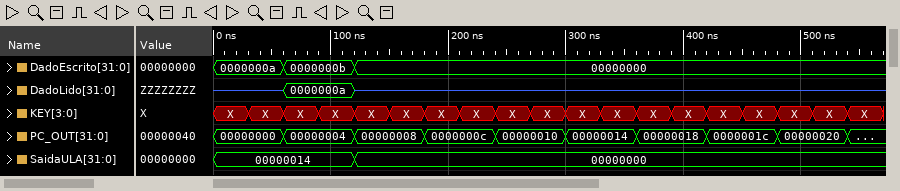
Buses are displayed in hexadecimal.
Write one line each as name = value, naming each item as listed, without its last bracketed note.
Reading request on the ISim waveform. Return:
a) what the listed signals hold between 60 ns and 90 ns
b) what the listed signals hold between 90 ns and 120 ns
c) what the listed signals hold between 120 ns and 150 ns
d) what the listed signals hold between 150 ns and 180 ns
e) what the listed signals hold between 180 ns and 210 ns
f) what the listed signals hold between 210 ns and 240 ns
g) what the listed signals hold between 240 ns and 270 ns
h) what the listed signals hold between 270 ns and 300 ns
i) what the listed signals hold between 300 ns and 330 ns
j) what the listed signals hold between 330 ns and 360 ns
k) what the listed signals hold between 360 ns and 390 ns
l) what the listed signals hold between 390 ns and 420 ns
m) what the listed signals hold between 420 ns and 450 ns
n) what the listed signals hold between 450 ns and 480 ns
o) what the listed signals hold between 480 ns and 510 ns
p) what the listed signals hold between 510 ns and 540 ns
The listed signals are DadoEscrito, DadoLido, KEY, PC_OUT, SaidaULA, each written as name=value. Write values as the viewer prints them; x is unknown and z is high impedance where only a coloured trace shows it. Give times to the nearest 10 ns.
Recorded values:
what the listed signals hold between 60 ns and 90 ns = DadoEscrito=0000000b, DadoLido=0000000a, KEY=X, PC_OUT=00000004, SaidaULA=00000014
what the listed signals hold between 90 ns and 120 ns = DadoEscrito=0000000b, DadoLido=0000000a, KEY=X, PC_OUT=00000004, SaidaULA=00000014
what the listed signals hold between 120 ns and 150 ns = DadoEscrito=00000000, DadoLido=z, KEY=X, PC_OUT=00000008, SaidaULA=00000000
what the listed signals hold between 150 ns and 180 ns = DadoEscrito=00000000, DadoLido=z, KEY=X, PC_OUT=00000008, SaidaULA=00000000
what the listed signals hold between 180 ns and 210 ns = DadoEscrito=00000000, DadoLido=z, KEY=X, PC_OUT=0000000c, SaidaULA=00000000
what the listed signals hold between 210 ns and 240 ns = DadoEscrito=00000000, DadoLido=z, KEY=X, PC_OUT=0000000c, SaidaULA=00000000
what the listed signals hold between 240 ns and 270 ns = DadoEscrito=00000000, DadoLido=z, KEY=X, PC_OUT=00000010, SaidaULA=00000000
what the listed signals hold between 270 ns and 300 ns = DadoEscrito=00000000, DadoLido=z, KEY=X, PC_OUT=00000010, SaidaULA=00000000
what the listed signals hold between 300 ns and 330 ns = DadoEscrito=00000000, DadoLido=z, KEY=X, PC_OUT=00000014, SaidaULA=00000000
what the listed signals hold between 330 ns and 360 ns = DadoEscrito=00000000, DadoLido=z, KEY=X, PC_OUT=00000014, SaidaULA=00000000
what the listed signals hold between 360 ns and 390 ns = DadoEscrito=00000000, DadoLido=z, KEY=X, PC_OUT=00000018, SaidaULA=00000000
what the listed signals hold between 390 ns and 420 ns = DadoEscrito=00000000, DadoLido=z, KEY=X, PC_OUT=00000018, SaidaULA=00000000
what the listed signals hold between 420 ns and 450 ns = DadoEscrito=00000000, DadoLido=z, KEY=X, PC_OUT=0000001c, SaidaULA=00000000
what the listed signals hold between 450 ns and 480 ns = DadoEscrito=00000000, DadoLido=z, KEY=X, PC_OUT=0000001c, SaidaULA=00000000
what the listed signals hold between 480 ns and 510 ns = DadoEscrito=00000000, DadoLido=z, KEY=X, PC_OUT=00000020, SaidaULA=00000000
what the listed signals hold between 510 ns and 540 ns = DadoEscrito=00000000, DadoLido=z, KEY=X, PC_OUT=00000020, SaidaULA=00000000
